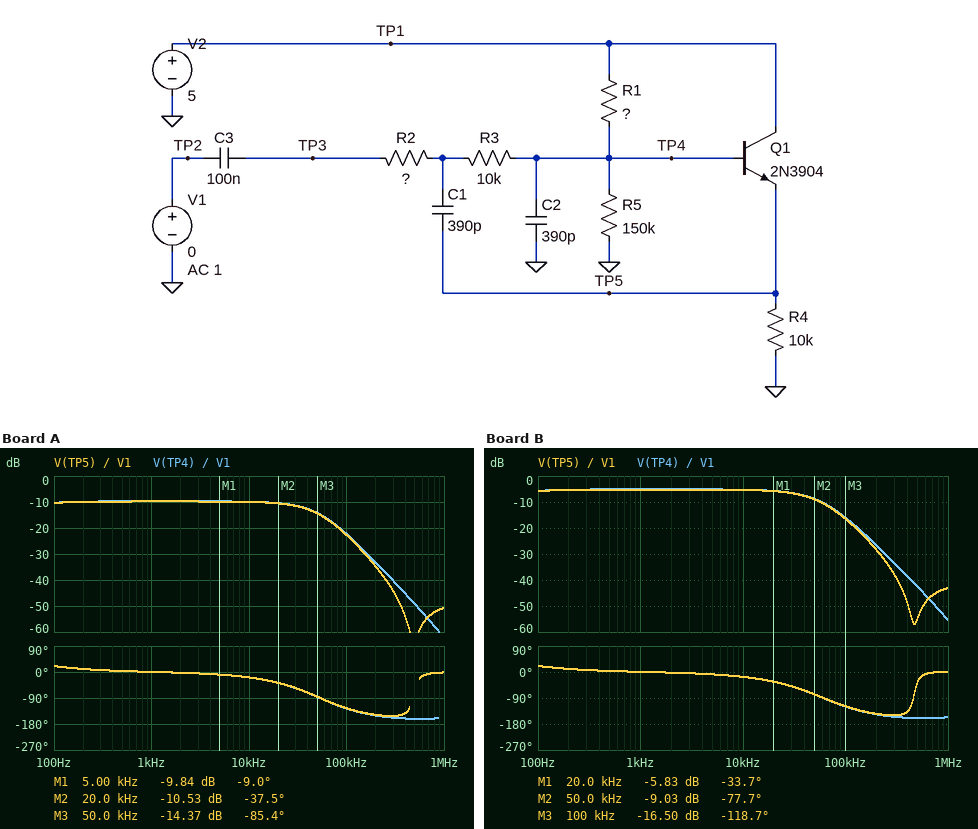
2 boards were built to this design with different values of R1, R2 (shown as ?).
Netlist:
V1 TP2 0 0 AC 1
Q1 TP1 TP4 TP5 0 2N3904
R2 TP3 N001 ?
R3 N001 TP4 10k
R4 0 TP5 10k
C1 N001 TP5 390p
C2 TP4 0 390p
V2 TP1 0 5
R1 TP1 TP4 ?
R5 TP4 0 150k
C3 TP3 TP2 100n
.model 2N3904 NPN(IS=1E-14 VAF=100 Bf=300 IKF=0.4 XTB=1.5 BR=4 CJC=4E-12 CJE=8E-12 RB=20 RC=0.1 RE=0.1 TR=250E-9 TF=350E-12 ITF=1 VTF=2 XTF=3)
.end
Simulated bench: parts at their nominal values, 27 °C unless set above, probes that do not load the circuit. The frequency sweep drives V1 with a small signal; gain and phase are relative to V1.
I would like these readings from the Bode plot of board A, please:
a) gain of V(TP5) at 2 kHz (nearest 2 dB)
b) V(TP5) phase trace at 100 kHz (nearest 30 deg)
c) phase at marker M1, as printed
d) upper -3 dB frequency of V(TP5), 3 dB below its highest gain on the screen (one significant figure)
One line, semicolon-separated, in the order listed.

-10 dB; -120 deg; -9.0 deg; 40 kHz
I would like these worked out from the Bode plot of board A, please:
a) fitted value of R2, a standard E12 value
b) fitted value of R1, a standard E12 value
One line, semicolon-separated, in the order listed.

18 kΩ; 15 kΩ
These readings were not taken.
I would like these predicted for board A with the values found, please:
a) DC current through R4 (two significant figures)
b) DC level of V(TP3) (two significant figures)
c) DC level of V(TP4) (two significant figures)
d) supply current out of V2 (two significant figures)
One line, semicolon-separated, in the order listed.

390 µA; 4.5 V; 4.5 V; 420 µA
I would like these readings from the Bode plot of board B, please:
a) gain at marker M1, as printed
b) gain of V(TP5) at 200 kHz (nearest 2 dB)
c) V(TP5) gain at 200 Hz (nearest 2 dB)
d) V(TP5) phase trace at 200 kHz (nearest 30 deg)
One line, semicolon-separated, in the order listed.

-5.83 dB; -28 dB; -6 dB; -150 deg
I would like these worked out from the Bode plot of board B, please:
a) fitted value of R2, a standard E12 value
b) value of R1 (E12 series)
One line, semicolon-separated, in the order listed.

8.2 kΩ; 27 kΩ
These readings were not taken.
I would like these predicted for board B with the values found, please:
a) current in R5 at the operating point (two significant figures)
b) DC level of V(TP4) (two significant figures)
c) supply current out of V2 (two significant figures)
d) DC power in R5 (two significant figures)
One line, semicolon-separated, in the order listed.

28 µA; 4.2 V; 390 µA; 120 µW
